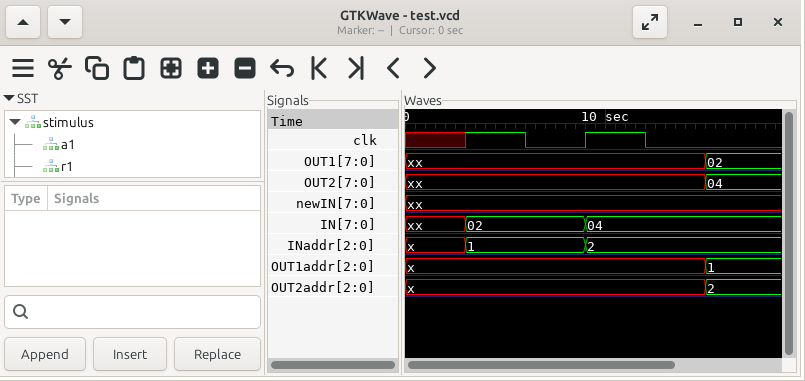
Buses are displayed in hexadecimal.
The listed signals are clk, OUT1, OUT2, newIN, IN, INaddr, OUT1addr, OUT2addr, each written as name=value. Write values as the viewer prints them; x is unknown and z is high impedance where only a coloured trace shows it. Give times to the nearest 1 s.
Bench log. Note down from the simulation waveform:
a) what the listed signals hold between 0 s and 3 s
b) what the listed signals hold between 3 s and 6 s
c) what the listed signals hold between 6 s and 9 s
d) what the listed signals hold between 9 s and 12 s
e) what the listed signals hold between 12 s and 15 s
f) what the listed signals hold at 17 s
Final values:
clk=x, OUT1=xx, OUT2=xx, newIN=xx, IN=xx, INaddr=x, OUT1addr=x, OUT2addr=x
clk=1, OUT1=xx, OUT2=xx, newIN=xx, IN=02, INaddr=1, OUT1addr=x, OUT2addr=x
clk=0, OUT1=xx, OUT2=xx, newIN=xx, IN=02, INaddr=1, OUT1addr=x, OUT2addr=x
clk=1, OUT1=xx, OUT2=xx, newIN=xx, IN=04, INaddr=2, OUT1addr=x, OUT2addr=x
clk=0, OUT1=xx, OUT2=xx, newIN=xx, IN=04, INaddr=2, OUT1addr=x, OUT2addr=x
clk=0, OUT1=02, OUT2=04, newIN=xx, IN=04, INaddr=2, OUT1addr=1, OUT2addr=2
